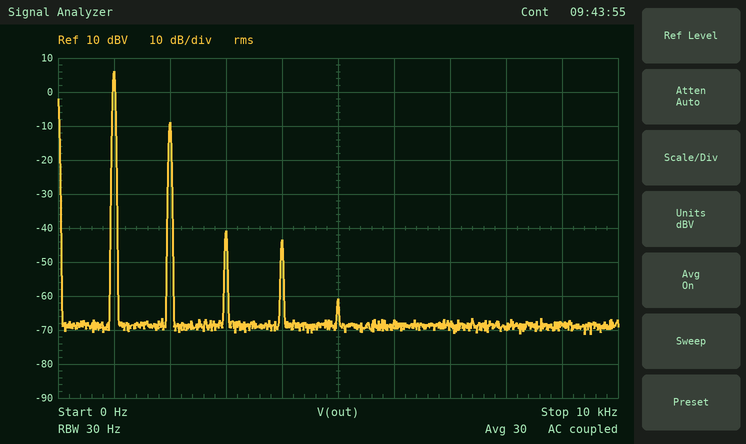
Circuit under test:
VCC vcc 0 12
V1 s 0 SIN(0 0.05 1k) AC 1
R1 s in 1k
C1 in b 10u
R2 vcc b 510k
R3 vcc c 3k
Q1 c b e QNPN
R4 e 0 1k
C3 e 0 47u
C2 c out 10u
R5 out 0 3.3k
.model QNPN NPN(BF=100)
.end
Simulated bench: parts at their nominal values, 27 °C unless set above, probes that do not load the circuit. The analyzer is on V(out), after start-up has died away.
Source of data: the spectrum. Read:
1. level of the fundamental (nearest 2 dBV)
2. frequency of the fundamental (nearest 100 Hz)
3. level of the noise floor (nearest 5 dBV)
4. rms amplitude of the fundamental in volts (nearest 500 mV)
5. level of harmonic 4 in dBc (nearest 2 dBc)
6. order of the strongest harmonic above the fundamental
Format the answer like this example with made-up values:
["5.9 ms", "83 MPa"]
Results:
["6 dBV", "1.0 kHz", "-70 dBV", "2.0 V", "-50 dBc", "2"]
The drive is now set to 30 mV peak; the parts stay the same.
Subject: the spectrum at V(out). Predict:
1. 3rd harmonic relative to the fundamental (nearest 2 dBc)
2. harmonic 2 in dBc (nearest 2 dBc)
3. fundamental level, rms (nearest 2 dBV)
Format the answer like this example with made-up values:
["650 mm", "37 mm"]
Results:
["-52 dBc", "-20 dBc", "2 dBV"]
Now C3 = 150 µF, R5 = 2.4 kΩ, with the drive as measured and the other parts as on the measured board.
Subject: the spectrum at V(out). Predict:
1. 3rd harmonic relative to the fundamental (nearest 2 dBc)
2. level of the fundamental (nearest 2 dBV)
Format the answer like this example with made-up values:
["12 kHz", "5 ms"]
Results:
["-52 dBc", "4 dBV"]
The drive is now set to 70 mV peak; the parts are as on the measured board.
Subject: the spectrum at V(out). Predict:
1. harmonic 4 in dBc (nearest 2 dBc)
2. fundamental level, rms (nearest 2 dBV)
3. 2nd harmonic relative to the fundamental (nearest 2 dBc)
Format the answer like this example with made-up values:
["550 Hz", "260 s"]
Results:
["-38 dBc", "8 dBV", "-12 dBc"]
